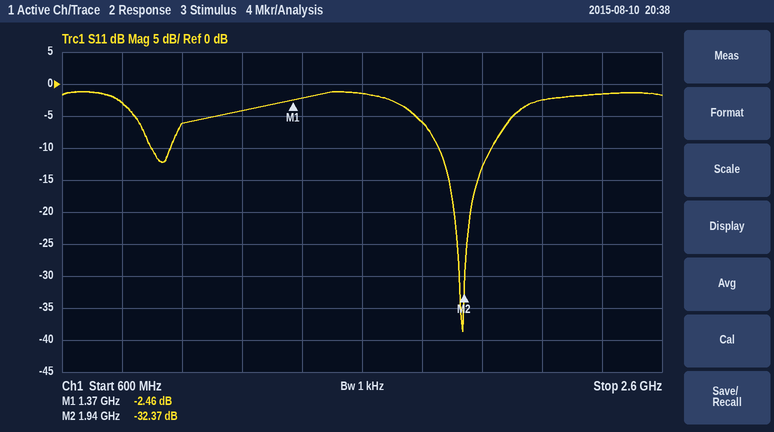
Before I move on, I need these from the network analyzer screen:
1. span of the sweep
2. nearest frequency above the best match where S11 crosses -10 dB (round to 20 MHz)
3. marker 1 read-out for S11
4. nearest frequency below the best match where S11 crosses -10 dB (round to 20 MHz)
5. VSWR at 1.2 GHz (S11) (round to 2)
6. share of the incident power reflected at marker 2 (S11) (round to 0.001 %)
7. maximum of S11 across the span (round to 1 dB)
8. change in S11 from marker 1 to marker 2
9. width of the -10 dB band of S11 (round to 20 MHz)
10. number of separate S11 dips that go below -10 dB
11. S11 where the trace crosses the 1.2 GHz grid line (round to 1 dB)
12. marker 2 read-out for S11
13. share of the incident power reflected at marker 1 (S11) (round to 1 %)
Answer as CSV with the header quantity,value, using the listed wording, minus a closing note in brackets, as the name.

quantity,value
span of the sweep,2 GHz
nearest frequency above the best match where S11 crosses -10 dB,2.04 GHz
marker 1 read-out for S11,-2.46 dB
nearest frequency below the best match where S11 crosses -10 dB,1.86 GHz
VSWR at 1.2 GHz (S11),4
share of the incident power reflected at marker 2 (S11),0.058 %
maximum of S11 across the span,-1 dB
change in S11 from marker 1 to marker 2,-29.91 dB
width of the -10 dB band of S11,180 MHz
number of separate S11 dips that go below -10 dB,2
S11 where the trace crosses the 1.2 GHz grid line,-4 dB
marker 2 read-out for S11,-32.37 dB
share of the incident power reflected at marker 1 (S11),57 %
